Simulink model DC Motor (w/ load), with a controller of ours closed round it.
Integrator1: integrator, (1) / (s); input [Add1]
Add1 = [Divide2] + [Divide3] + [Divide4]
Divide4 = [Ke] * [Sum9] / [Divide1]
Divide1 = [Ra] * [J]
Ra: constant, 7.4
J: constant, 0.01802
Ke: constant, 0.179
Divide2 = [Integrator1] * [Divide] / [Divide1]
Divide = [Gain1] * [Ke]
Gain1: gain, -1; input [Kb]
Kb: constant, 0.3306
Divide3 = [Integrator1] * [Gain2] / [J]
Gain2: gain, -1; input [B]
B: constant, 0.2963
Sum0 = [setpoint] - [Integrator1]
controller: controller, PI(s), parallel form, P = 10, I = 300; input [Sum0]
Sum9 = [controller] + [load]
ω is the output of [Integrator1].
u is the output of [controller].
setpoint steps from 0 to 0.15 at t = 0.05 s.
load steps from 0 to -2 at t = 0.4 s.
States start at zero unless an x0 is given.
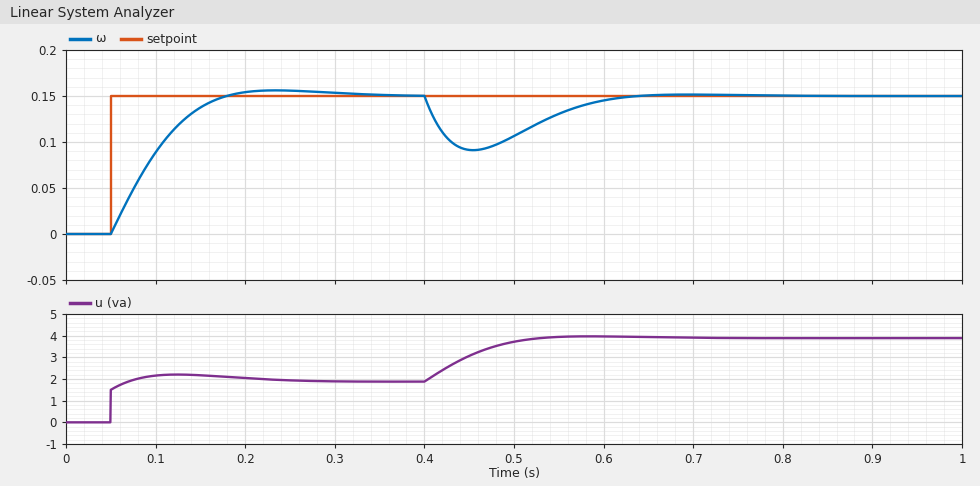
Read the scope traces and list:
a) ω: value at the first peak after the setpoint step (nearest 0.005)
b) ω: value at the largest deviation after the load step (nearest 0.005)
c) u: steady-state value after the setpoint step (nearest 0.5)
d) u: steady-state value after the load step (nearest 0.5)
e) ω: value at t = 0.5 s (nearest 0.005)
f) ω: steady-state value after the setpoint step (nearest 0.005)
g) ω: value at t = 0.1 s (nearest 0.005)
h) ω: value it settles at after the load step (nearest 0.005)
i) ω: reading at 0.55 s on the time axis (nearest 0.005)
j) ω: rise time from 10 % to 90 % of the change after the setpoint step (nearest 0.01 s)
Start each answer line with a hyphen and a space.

- 0.155
- 0.090
- 2.0
- 4.0
- 0.105
- 0.150
- 0.090
- 0.150
- 0.130
- 0.09 s
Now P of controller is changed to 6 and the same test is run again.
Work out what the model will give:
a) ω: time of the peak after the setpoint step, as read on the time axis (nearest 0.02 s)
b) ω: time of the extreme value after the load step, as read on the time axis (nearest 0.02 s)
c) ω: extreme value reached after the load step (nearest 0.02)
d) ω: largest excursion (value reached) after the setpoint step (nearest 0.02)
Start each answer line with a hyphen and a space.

- 0.22 s
- 0.46 s
- 0.08
- 0.16
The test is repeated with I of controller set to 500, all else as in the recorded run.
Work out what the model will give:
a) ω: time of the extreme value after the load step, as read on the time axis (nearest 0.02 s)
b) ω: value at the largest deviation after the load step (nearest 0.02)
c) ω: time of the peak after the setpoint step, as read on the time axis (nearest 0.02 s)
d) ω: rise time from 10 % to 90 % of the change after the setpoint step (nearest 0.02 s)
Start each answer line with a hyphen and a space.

- 0.44 s
- 0.10
- 0.18 s
- 0.06 s
